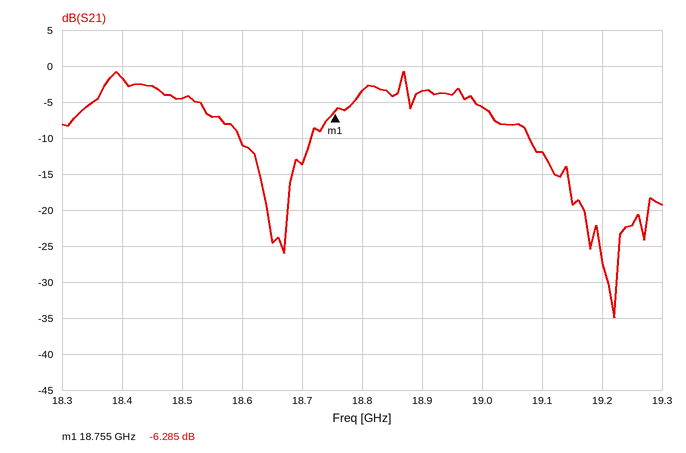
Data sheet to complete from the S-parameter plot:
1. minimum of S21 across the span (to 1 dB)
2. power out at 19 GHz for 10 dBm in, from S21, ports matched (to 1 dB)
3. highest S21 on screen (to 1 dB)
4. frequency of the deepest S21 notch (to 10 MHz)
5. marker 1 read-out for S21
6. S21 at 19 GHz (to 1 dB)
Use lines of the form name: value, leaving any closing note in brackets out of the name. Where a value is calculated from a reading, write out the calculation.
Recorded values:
minimum of S21 across the span: -35 dB
power out at 19 GHz for 10 dBm in, from S21, ports matched: 10 dBm + (-6 dB) = 4 dBm
highest S21 on screen: -1 dB
frequency of the deepest S21 notch: 19.22 GHz
marker 1 read-out for S21: -6.285 dB
S21 at 19 GHz: -6 dB
